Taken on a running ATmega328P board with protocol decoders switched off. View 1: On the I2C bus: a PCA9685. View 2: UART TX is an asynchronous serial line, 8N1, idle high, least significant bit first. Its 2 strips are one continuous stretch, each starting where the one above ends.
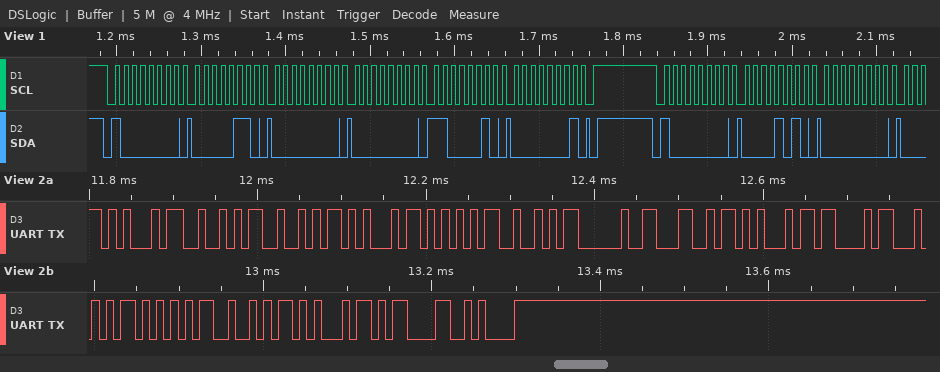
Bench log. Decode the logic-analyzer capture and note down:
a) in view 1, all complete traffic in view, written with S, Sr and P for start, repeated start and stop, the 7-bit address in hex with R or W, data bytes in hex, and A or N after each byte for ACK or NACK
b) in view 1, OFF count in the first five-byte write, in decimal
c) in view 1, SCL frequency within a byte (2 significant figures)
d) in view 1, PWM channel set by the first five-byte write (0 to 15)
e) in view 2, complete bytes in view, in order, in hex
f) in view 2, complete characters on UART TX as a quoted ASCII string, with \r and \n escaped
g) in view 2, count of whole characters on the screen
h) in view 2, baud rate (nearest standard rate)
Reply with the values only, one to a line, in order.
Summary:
S 40W A 06 A 00 A 00 A C2 A 01 A P S 40W A 0A A 00 A
450
100 kHz
0
45 52 52 45 55 52 20 4C 45 43 54 55 52 45 0D 0A
"ERREUR LECTURE\r\n"
16
115200 baud
